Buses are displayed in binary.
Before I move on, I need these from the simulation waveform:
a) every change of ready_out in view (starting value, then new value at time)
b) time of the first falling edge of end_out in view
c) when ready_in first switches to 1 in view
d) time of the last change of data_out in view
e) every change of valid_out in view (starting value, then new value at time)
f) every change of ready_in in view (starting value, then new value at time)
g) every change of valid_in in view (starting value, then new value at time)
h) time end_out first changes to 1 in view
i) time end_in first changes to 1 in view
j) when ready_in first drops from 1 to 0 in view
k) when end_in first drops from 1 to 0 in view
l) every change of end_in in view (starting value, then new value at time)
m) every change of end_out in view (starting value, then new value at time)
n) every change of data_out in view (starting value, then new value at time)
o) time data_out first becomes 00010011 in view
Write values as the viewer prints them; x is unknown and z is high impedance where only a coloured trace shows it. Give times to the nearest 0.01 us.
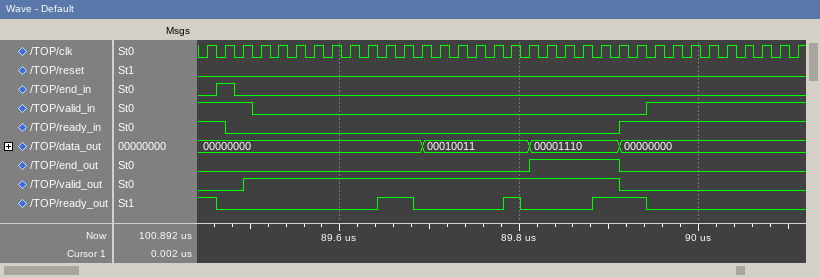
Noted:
1, 0 at 89.46 us, 1 at 89.64 us, 0 at 89.68 us, 1 at 89.78 us, 0 at 89.8 us, 1 at 89.88 us, 0 at 89.94 us
89.91 us
89.91 us
89.91 us
0, 1 at 89.49 us, 0 at 89.91 us
1, 0 at 89.47 us, 1 at 89.91 us
1, 0 at 89.5 us, 1 at 89.94 us
89.81 us
89.46 us
89.47 us
89.48 us
0, 1 at 89.46 us, 0 at 89.48 us
0, 1 at 89.81 us, 0 at 89.91 us
00000000, 00010011 at 89.69 us, 00001110 at 89.81 us, 00000000 at 89.91 us
89.69 us
